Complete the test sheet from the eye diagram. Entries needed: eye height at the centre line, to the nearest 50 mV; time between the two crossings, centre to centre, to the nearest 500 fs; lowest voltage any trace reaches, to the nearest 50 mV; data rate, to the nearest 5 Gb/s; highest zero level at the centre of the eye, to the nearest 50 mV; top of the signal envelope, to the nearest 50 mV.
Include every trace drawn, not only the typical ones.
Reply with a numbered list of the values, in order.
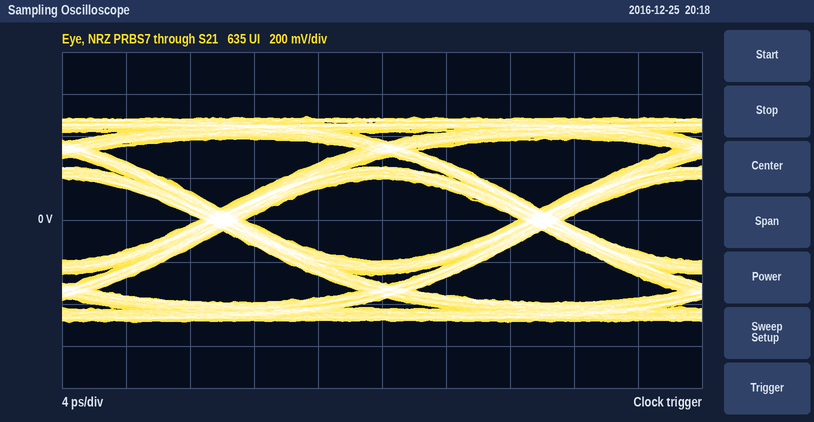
1. 400 mV
2. 20.0 ps
3. -500 mV
4. 50 Gb/s
5. -200 mV
6. 500 mV
